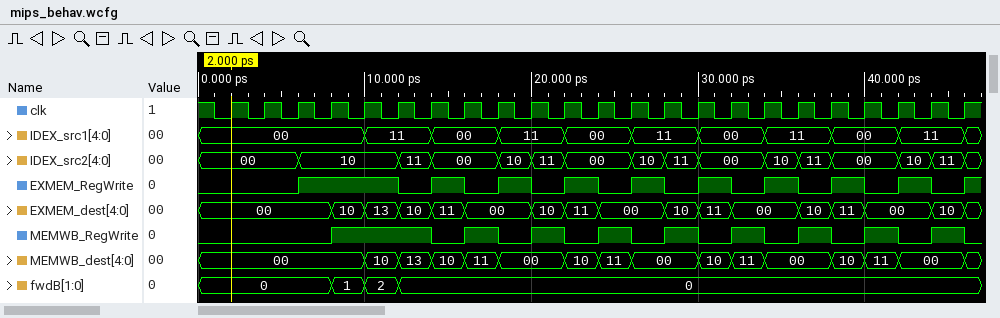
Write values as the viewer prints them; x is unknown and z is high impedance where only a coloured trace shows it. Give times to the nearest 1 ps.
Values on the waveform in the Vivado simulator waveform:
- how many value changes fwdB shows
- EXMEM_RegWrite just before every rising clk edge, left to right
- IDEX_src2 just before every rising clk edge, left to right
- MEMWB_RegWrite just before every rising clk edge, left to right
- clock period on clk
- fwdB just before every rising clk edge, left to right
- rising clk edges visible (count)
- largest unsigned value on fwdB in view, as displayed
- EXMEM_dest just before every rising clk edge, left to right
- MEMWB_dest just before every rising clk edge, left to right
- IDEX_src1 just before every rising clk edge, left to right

3
0 0 0 1 1 1 0 1 0 1 0 1 0 1 0 1 0 1 0 1 0 1 0
00, 00, 00, 10, 10, 10, 11, 00, 00, 10, 11, 00, 00, 10, 11, 00, 00, 10, 11, 00, 00, 10, 11
0 0 0 0 1 1 1 0 1 0 1 0 1 0 1 0 1 0 1 0 1 0 1
2 ps
0, 0, 0, 0, 1, 2, 0, 0, 0, 0, 0, 0, 0, 0, 0, 0, 0, 0, 0, 0, 0, 0, 0
23
2
00, 00, 00, 00, 10, 13, 10, 11, 00, 00, 10, 11, 00, 00, 10, 11, 00, 00, 10, 11, 00, 00, 10
00, 00, 00, 00, 00, 10, 13, 10, 11, 00, 00, 10, 11, 00, 00, 10, 11, 00, 00, 10, 11, 00, 00
00, 00, 00, 00, 00, 11, 11, 00, 00, 11, 11, 00, 00, 11, 11, 00, 00, 11, 11, 00, 00, 11, 11
